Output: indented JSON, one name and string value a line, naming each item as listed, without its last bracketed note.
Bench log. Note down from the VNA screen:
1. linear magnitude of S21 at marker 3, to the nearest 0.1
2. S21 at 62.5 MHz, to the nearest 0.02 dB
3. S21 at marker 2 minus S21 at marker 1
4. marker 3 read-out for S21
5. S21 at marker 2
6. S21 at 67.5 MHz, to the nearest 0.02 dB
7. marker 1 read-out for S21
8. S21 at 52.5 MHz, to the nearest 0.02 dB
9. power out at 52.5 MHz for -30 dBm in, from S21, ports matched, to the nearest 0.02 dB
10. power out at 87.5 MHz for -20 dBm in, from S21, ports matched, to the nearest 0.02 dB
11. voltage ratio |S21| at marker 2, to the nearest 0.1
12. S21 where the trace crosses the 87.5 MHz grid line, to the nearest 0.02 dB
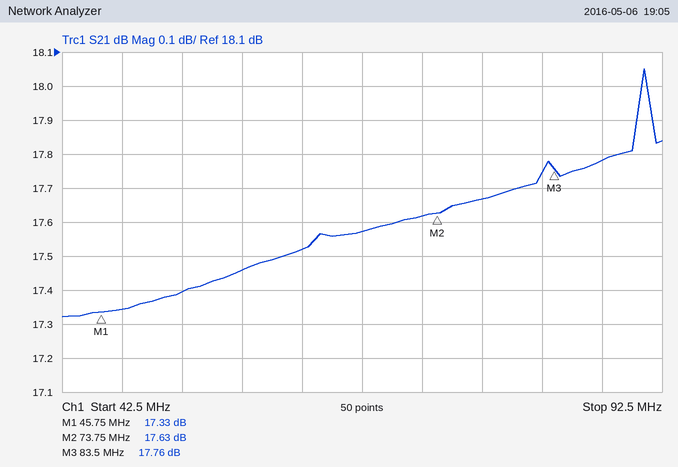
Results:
{
  "linear magnitude of S21 at marker 3, to the nearest 0.1": "7.7",
  "S21 at 62.5 MHz, to the nearest 0.02 dB": "17.52 dB",
  "S21 at marker 2 minus S21 at marker 1": "0.30 dB",
  "marker 3 read-out for S21": "17.76 dB",
  "S21 at marker 2": "17.63 dB",
  "S21 at 67.5 MHz, to the nearest 0.02 dB": "17.58 dB",
  "marker 1 read-out for S21": "17.33 dB",
  "S21 at 52.5 MHz, to the nearest 0.02 dB": "17.40 dB",
  "power out at 52.5 MHz for -30 dBm in, from S21, ports matched, to the nearest 0.02 dB": "-12.60 dBm",
  "power out at 87.5 MHz for -20 dBm in, from S21, ports matched, to the nearest 0.02 dB": "-2.22 dBm",
  "voltage ratio |S21| at marker 2, to the nearest 0.1": "7.6",
  "S21 where the trace crosses the 87.5 MHz grid line, to the nearest 0.02 dB": "17.78 dB"
}
